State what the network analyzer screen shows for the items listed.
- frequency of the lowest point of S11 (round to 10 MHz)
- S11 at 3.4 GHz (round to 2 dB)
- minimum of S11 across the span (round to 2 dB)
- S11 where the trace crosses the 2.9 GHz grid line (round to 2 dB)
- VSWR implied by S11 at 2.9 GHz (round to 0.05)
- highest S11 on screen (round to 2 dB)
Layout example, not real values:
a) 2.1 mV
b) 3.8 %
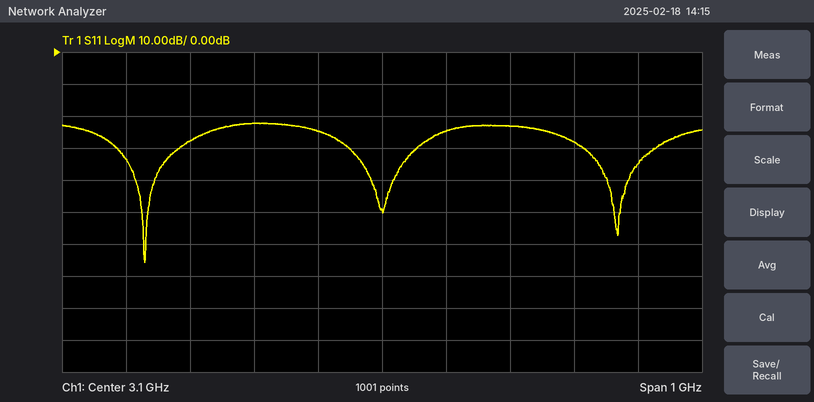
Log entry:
a) 2.73 GHz
b) -28 dB
c) -66 dB
d) -22 dB
e) 1.15
f) -22 dB
